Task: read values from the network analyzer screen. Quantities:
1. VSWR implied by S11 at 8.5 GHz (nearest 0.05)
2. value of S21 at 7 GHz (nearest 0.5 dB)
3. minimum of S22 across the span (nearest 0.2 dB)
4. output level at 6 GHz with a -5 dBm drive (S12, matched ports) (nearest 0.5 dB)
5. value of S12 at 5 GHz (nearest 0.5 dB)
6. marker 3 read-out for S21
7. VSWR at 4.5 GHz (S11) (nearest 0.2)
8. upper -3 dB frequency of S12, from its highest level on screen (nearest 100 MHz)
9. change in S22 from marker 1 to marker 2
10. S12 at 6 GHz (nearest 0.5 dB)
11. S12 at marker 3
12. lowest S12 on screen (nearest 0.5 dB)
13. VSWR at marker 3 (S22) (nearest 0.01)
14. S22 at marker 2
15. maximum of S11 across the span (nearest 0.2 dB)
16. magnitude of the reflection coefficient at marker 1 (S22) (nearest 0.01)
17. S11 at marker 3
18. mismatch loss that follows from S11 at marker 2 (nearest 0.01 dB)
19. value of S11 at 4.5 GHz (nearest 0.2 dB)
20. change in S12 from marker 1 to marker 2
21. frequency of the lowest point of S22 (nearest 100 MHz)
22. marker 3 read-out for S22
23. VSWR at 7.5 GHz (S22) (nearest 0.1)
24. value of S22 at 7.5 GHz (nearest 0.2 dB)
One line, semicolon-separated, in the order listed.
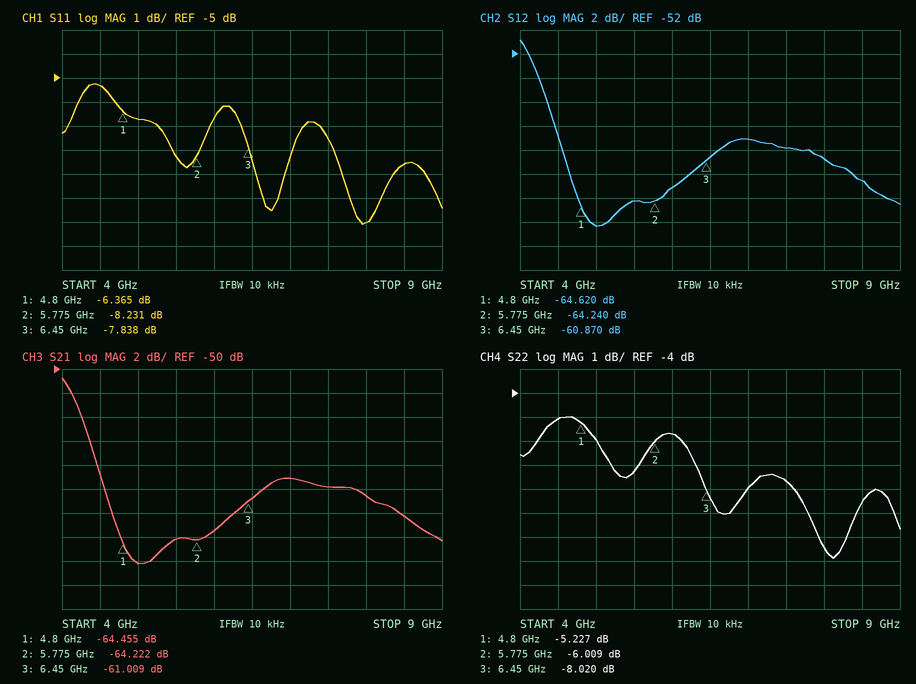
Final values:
2.20; -59.0 dB; -10.8 dB; -68.0 dBm; -66.5 dB; -61.009 dB; 3.4; 4.2 GHz; -0.782 dB; -63.0 dB; -60.870 dB; -66.5 dB; 2.32; -6.009 dB; -5.2 dB; 0.55; -7.838 dB; 0.71 dB; -5.4 dB; 0.380 dB; 8.1 GHz; -8.020 dB; 2.4; -7.6 dB
